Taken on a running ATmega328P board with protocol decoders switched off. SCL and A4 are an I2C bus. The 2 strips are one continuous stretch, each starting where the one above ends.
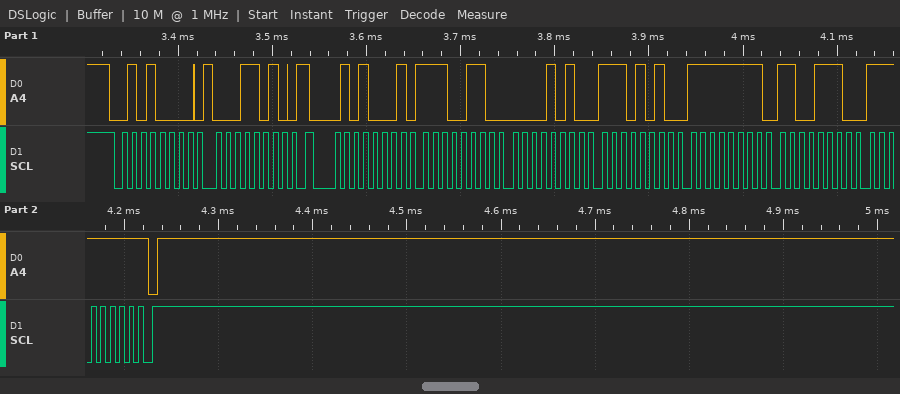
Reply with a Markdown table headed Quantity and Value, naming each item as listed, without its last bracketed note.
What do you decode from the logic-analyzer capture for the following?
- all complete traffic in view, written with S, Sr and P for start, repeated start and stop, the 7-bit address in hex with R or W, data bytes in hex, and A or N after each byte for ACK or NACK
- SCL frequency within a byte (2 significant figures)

| Quantity | Value |
|---|---|
| all complete traffic in view, written with S, Sr and P for start, repeated start and stop, the 7-bit address in hex with R or W, data bytes in hex, and A or N after each byte for ACK or NACK | S 28W A 1A A Sr 28R A E6 A 0A A EA A FF A CE A FF N P |
| SCL frequency within a byte | 100 kHz |
